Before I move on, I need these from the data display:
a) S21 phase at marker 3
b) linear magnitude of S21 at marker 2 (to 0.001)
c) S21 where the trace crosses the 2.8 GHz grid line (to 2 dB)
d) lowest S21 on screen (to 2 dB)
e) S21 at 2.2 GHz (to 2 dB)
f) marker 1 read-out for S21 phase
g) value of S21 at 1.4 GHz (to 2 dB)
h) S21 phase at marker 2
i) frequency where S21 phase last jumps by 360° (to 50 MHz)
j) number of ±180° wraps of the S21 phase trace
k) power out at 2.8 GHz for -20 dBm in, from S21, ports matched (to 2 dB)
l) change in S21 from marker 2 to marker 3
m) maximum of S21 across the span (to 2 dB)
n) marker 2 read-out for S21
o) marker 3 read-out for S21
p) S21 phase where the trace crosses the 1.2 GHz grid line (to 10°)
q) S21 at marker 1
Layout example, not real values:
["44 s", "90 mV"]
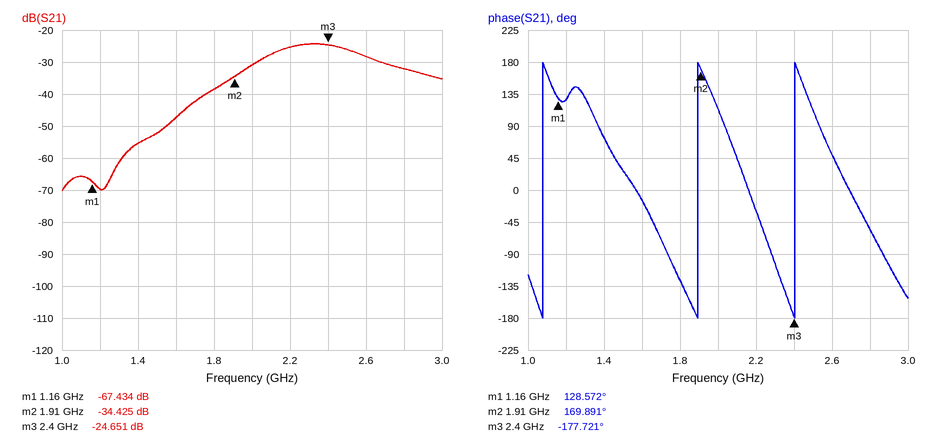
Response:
["-177.721°", "0.019", "-32 dB", "-70 dB", "-26 dB", "128.572°", "-56 dB", "169.891°", "2.40 GHz", "3", "-52 dBm", "9.774 dB", "-24 dB", "-34.425 dB", "-24.651 dB", "130°", "-67.434 dB"]
